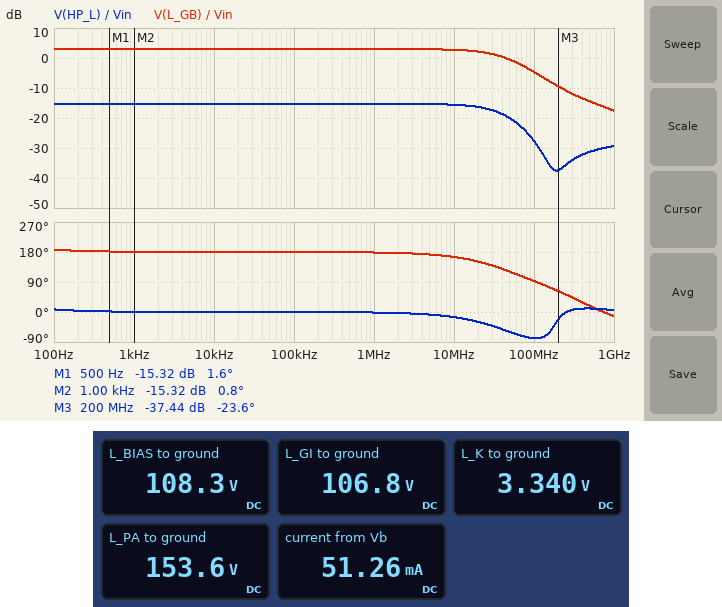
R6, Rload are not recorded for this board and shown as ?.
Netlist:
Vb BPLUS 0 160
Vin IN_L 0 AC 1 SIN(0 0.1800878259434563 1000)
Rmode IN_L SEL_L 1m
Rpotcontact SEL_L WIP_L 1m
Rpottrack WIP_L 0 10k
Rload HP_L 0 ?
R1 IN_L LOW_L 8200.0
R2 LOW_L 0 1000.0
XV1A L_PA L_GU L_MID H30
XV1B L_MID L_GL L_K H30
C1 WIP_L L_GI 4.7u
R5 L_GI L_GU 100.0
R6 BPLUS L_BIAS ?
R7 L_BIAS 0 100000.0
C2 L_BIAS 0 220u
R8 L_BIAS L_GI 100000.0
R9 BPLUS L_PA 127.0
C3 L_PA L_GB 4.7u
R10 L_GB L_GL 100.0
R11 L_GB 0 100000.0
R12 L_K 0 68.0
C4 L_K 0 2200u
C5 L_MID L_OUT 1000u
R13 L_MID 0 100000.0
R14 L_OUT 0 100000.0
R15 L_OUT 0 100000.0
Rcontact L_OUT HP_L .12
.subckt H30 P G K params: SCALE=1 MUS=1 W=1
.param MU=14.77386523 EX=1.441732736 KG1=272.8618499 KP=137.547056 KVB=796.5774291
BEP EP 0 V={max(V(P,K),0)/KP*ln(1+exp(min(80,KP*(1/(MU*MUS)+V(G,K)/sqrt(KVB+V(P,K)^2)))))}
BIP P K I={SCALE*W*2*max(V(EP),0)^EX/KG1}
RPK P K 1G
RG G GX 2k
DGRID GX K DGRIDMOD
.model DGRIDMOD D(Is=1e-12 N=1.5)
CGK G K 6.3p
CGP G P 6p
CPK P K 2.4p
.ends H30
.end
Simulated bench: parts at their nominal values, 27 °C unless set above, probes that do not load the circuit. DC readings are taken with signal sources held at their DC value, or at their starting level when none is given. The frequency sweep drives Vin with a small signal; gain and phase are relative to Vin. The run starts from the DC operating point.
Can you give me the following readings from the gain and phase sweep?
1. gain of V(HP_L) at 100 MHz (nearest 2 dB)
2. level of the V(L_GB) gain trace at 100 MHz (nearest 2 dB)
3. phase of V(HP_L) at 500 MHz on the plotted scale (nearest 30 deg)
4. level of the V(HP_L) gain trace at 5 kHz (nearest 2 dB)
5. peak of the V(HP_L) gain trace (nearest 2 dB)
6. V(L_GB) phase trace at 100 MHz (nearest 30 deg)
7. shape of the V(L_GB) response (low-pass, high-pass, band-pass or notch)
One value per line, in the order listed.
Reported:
-28 dB
-4 dB
0 deg
-16 dB
-16 dB
90 deg
low-pass
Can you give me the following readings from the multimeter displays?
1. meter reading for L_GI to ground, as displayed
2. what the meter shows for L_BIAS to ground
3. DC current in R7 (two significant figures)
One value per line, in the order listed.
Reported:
106.8 V
108.3 V
1.1 mA
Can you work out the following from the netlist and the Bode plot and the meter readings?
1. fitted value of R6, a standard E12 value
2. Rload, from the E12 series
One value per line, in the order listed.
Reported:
47 kΩ
4.7 Ω
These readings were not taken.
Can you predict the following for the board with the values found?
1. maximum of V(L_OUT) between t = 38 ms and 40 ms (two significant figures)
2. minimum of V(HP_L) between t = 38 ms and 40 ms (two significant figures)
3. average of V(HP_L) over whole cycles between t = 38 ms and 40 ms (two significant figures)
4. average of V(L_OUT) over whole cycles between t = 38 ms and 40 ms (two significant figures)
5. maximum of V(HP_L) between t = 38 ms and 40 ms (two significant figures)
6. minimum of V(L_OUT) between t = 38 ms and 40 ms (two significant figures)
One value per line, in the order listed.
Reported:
28 mV
-34 mV
-3.2 mV
-3.3 mV
28 mV
-35 mV
